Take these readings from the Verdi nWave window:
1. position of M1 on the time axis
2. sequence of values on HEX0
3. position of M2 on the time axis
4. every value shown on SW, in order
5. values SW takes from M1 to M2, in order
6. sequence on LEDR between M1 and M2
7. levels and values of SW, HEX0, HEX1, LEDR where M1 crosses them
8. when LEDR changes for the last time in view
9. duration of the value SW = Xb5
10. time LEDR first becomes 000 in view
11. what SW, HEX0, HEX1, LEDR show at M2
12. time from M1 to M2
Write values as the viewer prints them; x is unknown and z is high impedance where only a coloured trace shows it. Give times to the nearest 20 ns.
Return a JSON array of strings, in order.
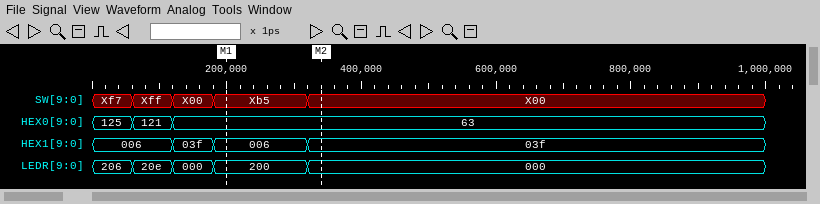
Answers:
["200 ns", "125, 121, 63", "340 ns", "Xf7, Xff, X00, Xb5, X00", "Xb5, X00", "200, 000", "SW=Xb5, HEX0=63, HEX1=006, LEDR=200", "320 ns", "140 ns", "120 ns", "SW=X00, HEX0=63, HEX1=03f, LEDR=000", "140 ns"]
